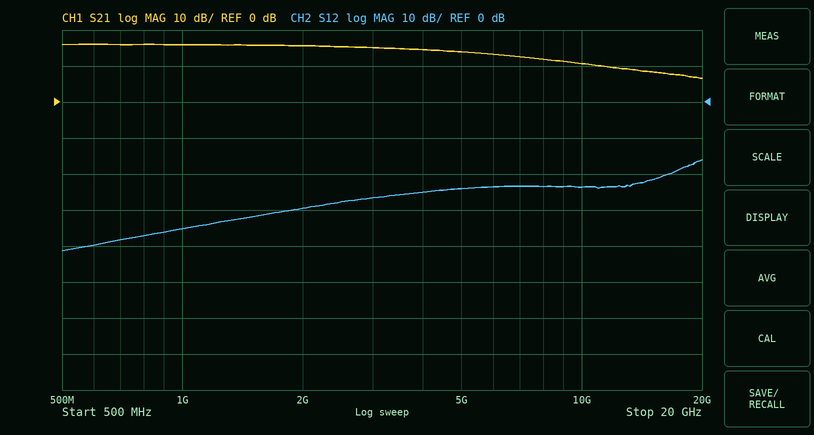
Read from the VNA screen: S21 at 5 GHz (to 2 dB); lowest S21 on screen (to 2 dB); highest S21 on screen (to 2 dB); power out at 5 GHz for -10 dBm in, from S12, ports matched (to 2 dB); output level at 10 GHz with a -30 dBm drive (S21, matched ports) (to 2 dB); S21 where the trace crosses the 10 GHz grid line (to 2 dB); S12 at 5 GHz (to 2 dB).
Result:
14 dB
6 dB
16 dB
-34 dBm
-20 dBm
10 dB
-24 dB
